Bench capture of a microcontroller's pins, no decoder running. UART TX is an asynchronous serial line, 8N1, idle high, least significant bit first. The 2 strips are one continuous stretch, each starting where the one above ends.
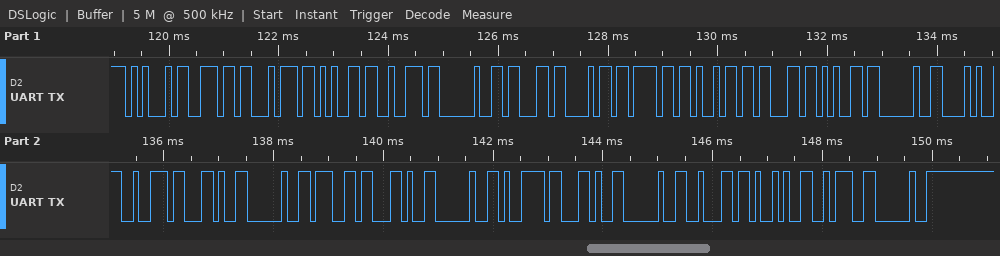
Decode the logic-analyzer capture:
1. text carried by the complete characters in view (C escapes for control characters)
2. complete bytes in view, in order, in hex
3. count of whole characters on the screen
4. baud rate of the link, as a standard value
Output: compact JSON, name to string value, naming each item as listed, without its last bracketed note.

{"text carried by the complete characters in view": "\"Enter choice (r, g, y, b): \"", "complete bytes in view, in order, in hex": "45 6E 74 65 72 20 63 68 6F 69 63 65 20 28 72 2C 20 67 2C 20 79 2C 20 62 29 3A 20", "count of whole characters on the screen": "27", "baud rate of the link, as a standard value": "9600 baud"}
